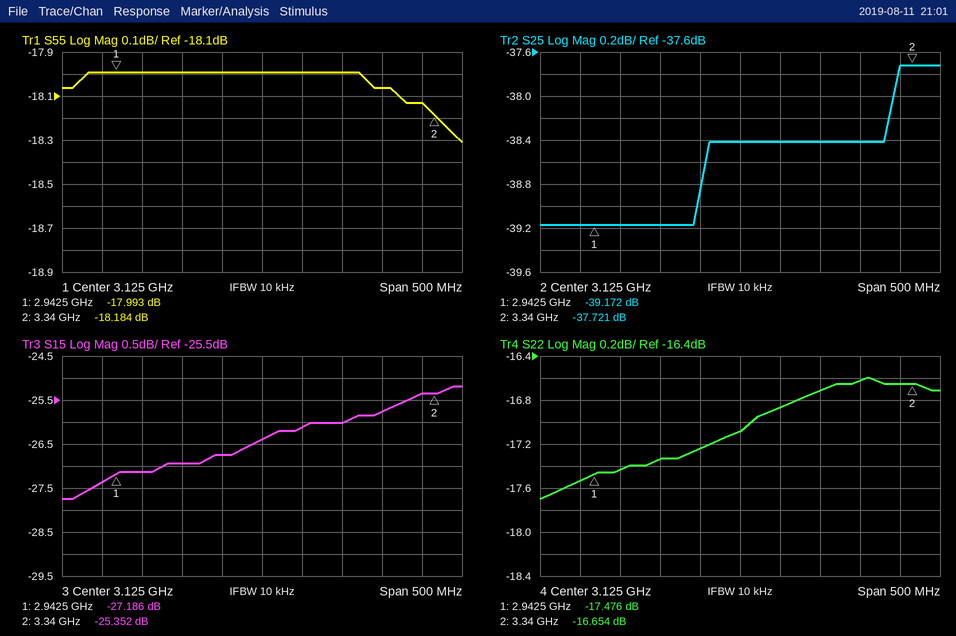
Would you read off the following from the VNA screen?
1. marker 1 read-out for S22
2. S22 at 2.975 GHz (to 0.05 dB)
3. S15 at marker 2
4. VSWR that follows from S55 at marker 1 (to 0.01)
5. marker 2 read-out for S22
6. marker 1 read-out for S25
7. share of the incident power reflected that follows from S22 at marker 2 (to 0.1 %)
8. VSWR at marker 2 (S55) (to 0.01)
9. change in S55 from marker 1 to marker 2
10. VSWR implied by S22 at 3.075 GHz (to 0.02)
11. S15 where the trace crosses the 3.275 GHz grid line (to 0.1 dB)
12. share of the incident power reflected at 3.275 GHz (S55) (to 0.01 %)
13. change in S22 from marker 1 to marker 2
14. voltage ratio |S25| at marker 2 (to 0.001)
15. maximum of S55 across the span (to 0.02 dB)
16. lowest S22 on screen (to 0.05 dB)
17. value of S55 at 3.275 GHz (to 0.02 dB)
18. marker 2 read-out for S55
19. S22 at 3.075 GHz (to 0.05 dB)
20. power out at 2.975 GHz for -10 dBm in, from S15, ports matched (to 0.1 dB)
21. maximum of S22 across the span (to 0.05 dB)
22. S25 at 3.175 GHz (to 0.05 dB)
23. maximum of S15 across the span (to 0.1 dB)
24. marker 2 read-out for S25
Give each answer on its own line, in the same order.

-17.476 dB
-17.45 dB
-25.352 dB
1.29
-16.654 dB
-39.172 dB
2.2 %
1.28
-0.191 dB
1.32
-25.8 dB
1.56 %
0.822 dB
0.013
-18.00 dB
-17.70 dB
-18.06 dB
-18.184 dB
-17.25 dB
-37.1 dBm
-16.60 dB
-38.40 dB
-25.2 dB
-37.721 dB
